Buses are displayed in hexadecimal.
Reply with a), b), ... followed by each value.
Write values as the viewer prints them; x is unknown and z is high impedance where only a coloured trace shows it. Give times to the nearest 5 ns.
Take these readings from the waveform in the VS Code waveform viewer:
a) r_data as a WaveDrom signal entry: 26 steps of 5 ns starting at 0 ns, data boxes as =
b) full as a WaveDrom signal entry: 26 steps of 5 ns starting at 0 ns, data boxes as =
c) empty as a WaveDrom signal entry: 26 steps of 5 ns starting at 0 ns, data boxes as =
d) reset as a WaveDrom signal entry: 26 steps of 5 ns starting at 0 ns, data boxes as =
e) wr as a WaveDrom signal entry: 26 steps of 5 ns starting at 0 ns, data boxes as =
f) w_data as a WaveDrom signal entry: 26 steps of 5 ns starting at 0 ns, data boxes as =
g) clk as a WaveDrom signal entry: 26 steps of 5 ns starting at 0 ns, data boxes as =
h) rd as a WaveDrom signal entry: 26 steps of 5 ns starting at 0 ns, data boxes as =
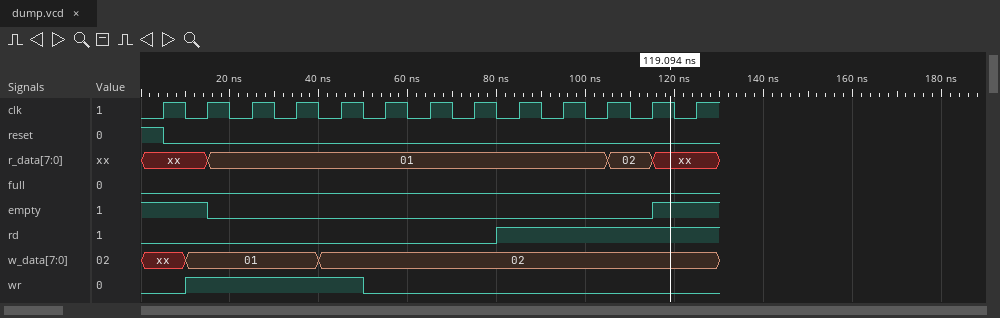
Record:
a) {name: 'r_data', wave: 'x..=.................=.x..', data: '01 02'}
b) {name: 'full', wave: '0.........................'}
c) {name: 'empty', wave: '1..0...................1..'}
d) {name: 'reset', wave: '10........................'}
e) {name: 'wr', wave: '0.1.......0...............'}
f) {name: 'w_data', wave: 'x.=.....=.................', data: '01 02'}
g) {name: 'clk', wave: '01010101010101010101010101'}
h) {name: 'rd', wave: '0...............1.........'}
